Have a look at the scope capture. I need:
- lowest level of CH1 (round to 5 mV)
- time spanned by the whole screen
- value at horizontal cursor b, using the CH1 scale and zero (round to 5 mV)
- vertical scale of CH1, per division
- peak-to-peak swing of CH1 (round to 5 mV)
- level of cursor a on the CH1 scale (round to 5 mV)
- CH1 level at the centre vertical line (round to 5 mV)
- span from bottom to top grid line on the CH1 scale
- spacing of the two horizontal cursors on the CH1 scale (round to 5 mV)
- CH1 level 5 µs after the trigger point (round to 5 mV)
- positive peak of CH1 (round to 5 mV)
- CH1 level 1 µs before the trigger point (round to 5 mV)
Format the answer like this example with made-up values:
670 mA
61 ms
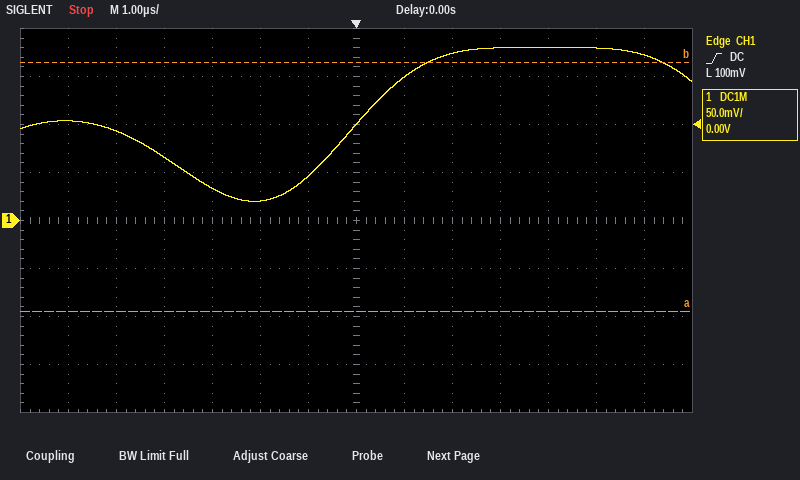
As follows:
20 mV
14 µs
165 mV
50 mV
160 mV
-95 mV
100 mV
400 mV
260 mV
180 mV
180 mV
45 mV
